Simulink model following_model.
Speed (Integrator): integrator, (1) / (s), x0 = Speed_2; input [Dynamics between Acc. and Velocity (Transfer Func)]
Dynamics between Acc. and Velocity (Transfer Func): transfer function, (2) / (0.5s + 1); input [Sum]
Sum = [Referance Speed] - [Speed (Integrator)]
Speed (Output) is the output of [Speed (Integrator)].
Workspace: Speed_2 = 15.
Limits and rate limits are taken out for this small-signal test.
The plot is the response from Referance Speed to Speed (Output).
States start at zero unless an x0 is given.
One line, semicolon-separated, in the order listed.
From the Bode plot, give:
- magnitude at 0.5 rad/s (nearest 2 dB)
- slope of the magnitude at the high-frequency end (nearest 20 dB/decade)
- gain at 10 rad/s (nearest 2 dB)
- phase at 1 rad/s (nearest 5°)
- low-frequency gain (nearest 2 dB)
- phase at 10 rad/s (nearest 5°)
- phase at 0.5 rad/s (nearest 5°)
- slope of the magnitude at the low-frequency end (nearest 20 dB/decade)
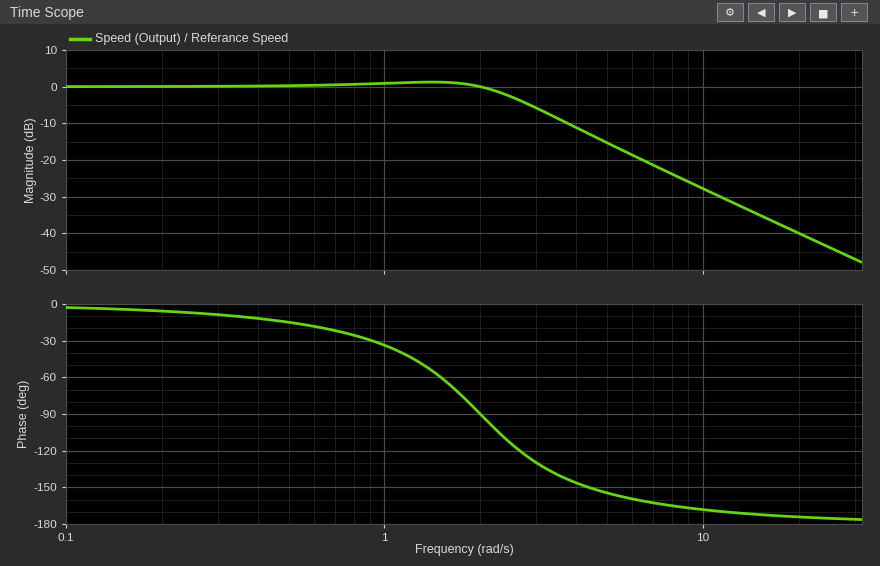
0 dB; -40 dB/decade; -28 dB; -35°; 0 dB; -170°; -15°; 0 dB/decade
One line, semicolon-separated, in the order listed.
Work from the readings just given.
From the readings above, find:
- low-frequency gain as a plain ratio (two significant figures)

1.0
